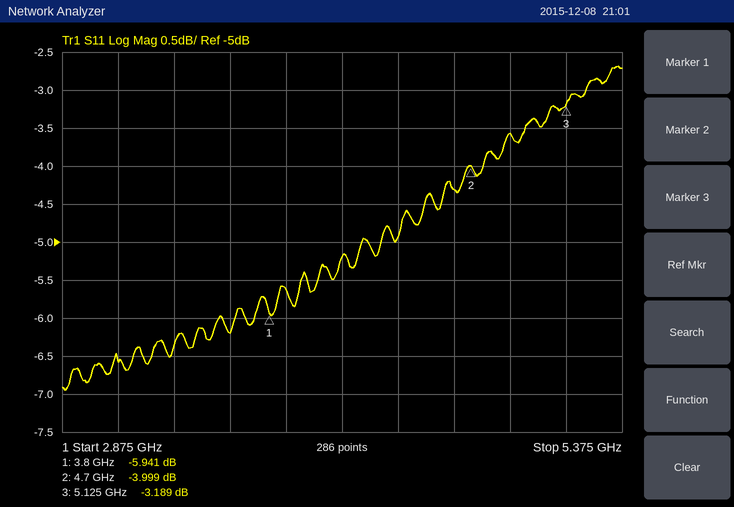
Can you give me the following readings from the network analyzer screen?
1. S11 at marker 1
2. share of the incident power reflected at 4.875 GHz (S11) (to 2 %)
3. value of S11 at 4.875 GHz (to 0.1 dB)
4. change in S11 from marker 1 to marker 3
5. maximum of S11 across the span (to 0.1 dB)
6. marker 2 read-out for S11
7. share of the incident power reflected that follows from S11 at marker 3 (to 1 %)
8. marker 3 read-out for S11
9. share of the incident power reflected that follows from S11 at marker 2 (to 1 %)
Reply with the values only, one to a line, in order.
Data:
-5.941 dB
44 %
-3.6 dB
2.752 dB
-2.7 dB
-3.999 dB
48 %
-3.189 dB
40 %
